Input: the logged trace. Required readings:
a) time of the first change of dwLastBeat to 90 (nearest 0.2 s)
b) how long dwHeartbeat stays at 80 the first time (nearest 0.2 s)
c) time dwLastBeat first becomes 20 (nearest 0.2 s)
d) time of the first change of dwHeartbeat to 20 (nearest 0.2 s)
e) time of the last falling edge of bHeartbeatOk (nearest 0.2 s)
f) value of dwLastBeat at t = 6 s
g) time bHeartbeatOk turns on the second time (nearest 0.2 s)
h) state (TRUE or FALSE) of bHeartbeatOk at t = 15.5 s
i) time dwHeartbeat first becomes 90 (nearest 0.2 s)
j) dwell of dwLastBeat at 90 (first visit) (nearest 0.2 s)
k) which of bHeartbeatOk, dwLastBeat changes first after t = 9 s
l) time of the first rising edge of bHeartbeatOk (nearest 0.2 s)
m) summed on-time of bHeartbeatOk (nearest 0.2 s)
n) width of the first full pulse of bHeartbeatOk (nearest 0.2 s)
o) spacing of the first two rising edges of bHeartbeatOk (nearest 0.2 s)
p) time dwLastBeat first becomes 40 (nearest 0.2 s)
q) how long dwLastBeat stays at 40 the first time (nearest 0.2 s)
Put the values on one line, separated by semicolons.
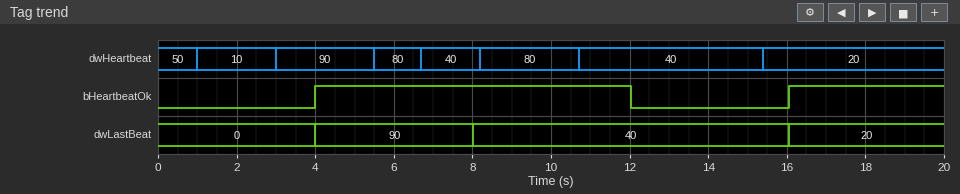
4.0 s; 1.2 s; 16.0 s; 15.4 s; 12.0 s; 90; 16.0 s; FALSE; 3.0 s; 4.0 s; bHeartbeatOk; 4.0 s; 12.0 s; 8.0 s; 12.0 s; 8.0 s; 8.0 s
